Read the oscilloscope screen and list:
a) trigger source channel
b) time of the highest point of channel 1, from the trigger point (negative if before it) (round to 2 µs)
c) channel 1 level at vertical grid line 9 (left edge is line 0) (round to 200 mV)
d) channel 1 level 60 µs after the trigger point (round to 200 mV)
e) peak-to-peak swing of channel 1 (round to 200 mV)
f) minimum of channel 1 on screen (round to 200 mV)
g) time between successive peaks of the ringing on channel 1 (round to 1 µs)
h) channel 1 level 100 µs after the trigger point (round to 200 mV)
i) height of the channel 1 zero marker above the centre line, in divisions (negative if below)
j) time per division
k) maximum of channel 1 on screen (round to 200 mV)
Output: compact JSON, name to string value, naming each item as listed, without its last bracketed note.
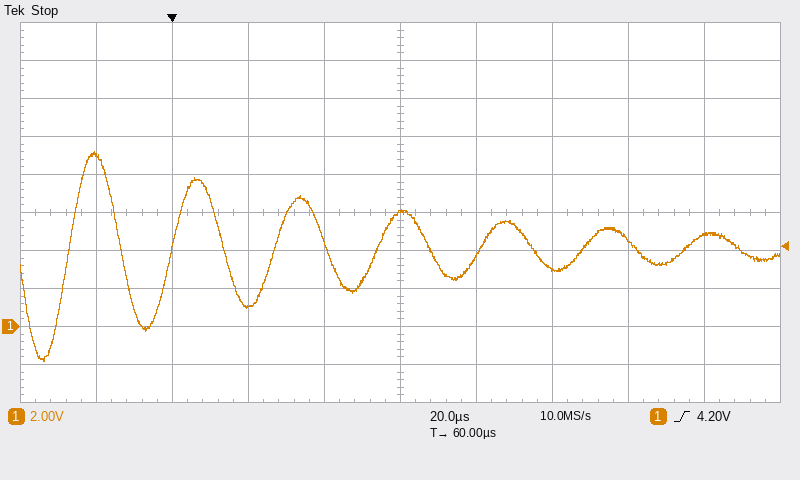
{"trigger source channel": "channel 1", "time of the highest point of channel 1, from the trigger point (negative if before it)": "-20 µs", "channel 1 level at vertical grid line 9 (left edge is line 0)": "4.8 V", "channel 1 level 60 µs after the trigger point": "6.0 V", "peak-to-peak swing of channel 1": "11.0 V", "minimum of channel 1 on screen": "-1.8 V", "time between successive peaks of the ringing on channel 1": "27 µs", "channel 1 level 100 µs after the trigger point": "3.0 V", "height of the channel 1 zero marker above the centre line, in divisions": "-3.0 div", "time per division": "20 µs", "maximum of channel 1 on screen": "9.2 V"}
